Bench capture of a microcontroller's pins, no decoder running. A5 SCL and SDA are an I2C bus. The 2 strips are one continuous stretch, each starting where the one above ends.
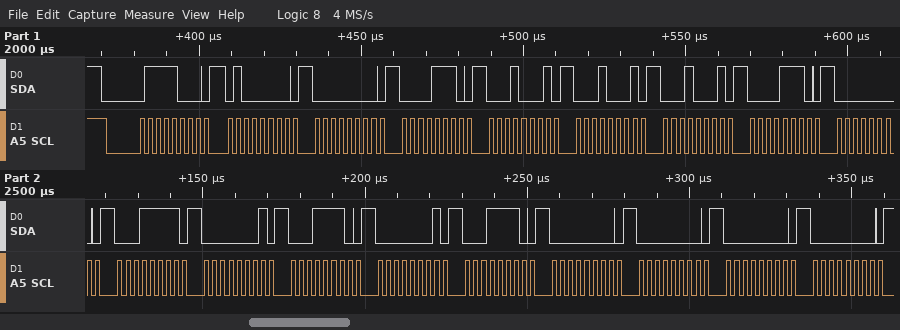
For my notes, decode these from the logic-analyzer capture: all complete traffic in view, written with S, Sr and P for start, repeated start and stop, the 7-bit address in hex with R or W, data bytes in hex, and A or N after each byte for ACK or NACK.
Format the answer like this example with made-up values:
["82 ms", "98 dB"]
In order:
["S 3CW A 40 A 00 A 0E A 11 A 11 A 11 A 0E A 00 A 1F A 01 A 1E A 01 A 1E A 00 A 00 A 00 A 00 A"]
